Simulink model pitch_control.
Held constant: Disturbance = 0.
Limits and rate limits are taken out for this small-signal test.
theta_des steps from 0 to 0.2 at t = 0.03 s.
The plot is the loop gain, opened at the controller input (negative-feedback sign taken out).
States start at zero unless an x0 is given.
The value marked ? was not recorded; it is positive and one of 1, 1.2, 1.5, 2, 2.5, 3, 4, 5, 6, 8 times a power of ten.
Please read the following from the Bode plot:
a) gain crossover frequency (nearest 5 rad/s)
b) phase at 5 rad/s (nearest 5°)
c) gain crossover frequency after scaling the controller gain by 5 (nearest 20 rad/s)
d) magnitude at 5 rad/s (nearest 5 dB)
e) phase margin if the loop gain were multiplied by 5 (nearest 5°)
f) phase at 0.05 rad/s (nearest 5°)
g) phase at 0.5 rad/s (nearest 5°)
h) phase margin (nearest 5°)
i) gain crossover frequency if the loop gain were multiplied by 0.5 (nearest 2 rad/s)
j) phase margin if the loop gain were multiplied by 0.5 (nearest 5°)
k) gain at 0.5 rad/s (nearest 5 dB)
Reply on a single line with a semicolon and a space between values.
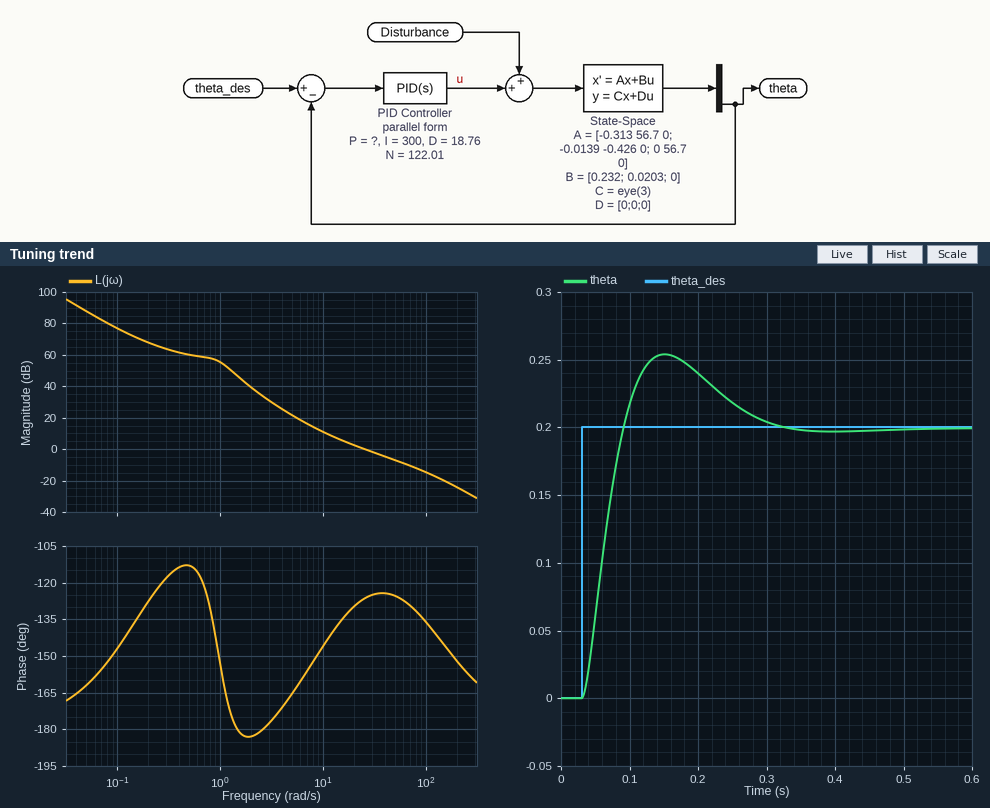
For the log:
25 rad/s; -165°; 100 rad/s; 20 dB; 45°; -160°; -115°; 55°; 14 rad/s; 45°; 60 dB
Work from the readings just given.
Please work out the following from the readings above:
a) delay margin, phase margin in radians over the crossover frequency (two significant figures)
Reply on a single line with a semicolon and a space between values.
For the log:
0.038 s
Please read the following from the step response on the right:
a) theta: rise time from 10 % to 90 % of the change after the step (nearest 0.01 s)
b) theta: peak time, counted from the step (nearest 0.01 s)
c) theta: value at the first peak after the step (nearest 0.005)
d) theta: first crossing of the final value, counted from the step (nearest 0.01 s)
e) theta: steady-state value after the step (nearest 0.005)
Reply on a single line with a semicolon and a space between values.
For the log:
0.04 s; 0.12 s; 0.255; 0.06 s; 0.200
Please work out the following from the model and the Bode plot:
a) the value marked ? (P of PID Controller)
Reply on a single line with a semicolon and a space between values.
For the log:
250
